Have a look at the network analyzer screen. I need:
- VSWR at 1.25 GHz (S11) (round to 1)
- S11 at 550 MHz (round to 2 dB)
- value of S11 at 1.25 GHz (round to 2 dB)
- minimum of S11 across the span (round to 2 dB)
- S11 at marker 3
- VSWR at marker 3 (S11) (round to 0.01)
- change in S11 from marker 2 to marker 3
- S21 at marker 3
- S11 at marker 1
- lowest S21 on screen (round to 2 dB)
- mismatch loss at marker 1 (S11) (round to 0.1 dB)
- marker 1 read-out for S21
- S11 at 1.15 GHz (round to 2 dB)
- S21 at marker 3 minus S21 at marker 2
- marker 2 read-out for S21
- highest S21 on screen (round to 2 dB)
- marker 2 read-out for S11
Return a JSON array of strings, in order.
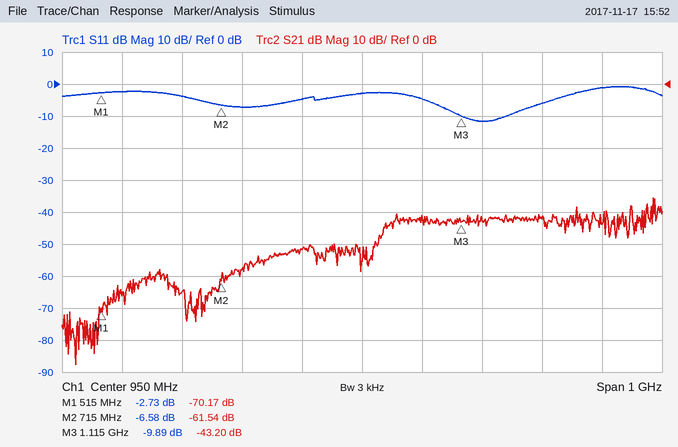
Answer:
["3", "-2 dB", "-6 dB", "-12 dB", "-9.89 dB", "1.94", "-3.31 dB", "-43.20 dB", "-2.73 dB", "-88 dB", "3.3 dB", "-70.17 dB", "-12 dB", "18.34 dB", "-61.54 dB", "-36 dB", "-6.58 dB"]
